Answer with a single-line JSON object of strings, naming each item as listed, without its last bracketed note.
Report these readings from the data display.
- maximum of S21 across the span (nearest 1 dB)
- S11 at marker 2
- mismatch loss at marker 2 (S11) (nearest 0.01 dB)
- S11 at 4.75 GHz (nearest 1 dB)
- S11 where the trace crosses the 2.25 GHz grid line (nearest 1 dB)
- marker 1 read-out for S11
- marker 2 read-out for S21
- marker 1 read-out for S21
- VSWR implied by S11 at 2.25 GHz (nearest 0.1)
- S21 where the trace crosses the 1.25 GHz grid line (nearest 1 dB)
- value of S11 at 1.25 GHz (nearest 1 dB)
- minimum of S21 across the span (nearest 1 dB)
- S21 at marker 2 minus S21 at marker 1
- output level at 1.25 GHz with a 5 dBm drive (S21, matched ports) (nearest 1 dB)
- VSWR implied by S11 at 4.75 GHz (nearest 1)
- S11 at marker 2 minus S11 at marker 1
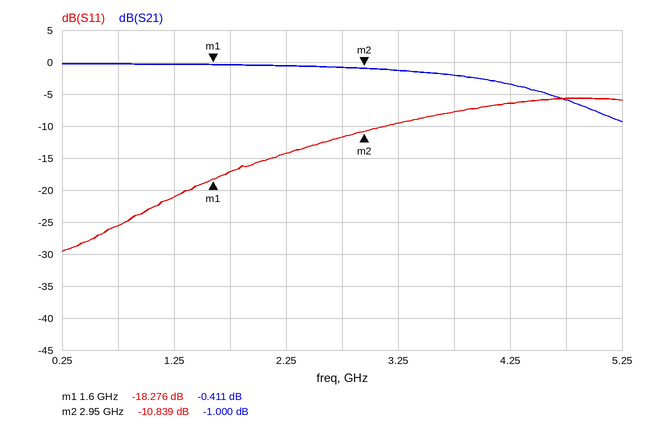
{"maximum of S21 across the span": "0 dB", "S11 at marker 2": "-10.839 dB", "mismatch loss at marker 2 (S11)": "0.37 dB", "S11 at 4.75 GHz": "-6 dB", "S11 where the trace crosses the 2.25 GHz grid line": "-14 dB", "marker 1 read-out for S11": "-18.276 dB", "marker 2 read-out for S21": "-1.000 dB", "marker 1 read-out for S21": "-0.411 dB", "VSWR implied by S11 at 2.25 GHz": "1.5", "S21 where the trace crosses the 1.25 GHz grid line": "0 dB", "value of S11 at 1.25 GHz": "-21 dB", "minimum of S21 across the span": "-9 dB", "S21 at marker 2 minus S21 at marker 1": "-0.589 dB", "output level at 1.25 GHz with a 5 dBm drive (S21, matched ports)": "5 dBm", "VSWR implied by S11 at 4.75 GHz": "3", "S11 at marker 2 minus S11 at marker 1": "7.437 dB"}
